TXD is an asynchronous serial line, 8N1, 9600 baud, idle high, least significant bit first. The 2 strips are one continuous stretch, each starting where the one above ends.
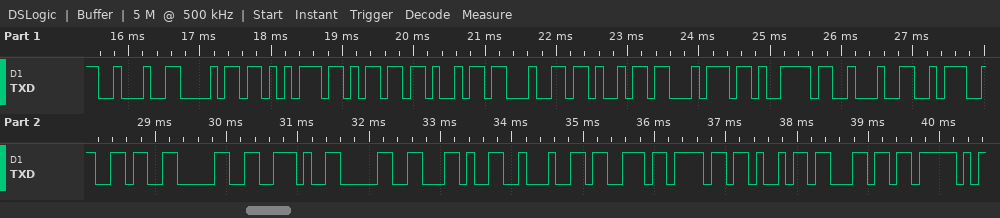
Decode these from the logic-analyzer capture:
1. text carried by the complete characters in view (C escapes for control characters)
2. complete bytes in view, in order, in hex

"\"humidity\":60.0,\"soil_"
22 68 75 6D 69 64 69 74 79 22 3A 36 30 2E 30 2C 22 73 6F 69 6C 5F
